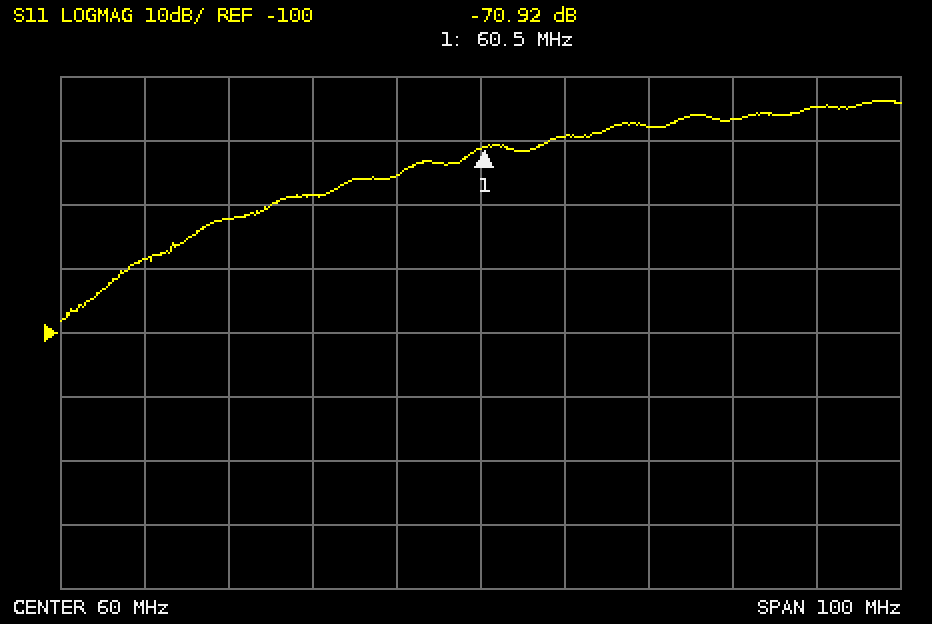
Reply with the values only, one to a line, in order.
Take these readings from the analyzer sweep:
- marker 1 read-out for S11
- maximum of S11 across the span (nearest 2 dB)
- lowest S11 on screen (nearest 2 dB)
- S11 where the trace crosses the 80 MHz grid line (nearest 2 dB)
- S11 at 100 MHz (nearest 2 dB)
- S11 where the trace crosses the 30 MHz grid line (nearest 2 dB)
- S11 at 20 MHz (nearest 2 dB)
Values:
-70.92 dB
-64 dB
-98 dB
-68 dB
-64 dB
-82 dB
-88 dB
